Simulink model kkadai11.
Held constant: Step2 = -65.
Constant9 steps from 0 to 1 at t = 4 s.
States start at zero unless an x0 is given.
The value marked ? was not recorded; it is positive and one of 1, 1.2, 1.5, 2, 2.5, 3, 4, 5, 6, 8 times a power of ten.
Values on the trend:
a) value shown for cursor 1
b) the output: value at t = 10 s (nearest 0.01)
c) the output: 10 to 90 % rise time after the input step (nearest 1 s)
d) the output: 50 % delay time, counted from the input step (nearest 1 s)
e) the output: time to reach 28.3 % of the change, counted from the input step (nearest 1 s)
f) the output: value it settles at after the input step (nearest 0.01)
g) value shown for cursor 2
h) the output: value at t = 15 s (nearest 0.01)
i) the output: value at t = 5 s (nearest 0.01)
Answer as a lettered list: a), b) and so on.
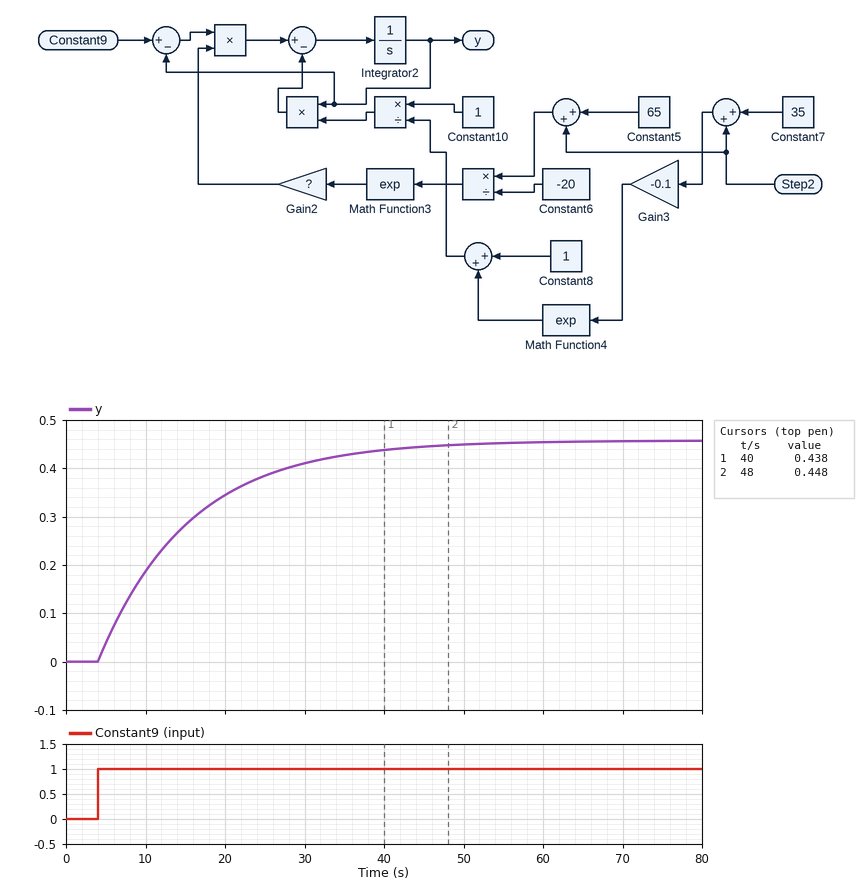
a) 0.438
b) 0.19
c) 25 s
d) 8 s
e) 4 s
f) 0.46
g) 0.448
h) 0.28
i) 0.04
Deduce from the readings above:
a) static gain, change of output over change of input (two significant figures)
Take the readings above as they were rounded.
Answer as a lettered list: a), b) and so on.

a) 0.46
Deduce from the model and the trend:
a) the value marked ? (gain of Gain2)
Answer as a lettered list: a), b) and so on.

a) 0.04
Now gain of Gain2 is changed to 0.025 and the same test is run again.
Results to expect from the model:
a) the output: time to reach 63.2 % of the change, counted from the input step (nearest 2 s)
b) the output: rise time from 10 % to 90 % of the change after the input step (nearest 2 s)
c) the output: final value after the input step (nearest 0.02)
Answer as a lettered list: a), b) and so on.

a) 14 s
b) 30 s
c) 0.34
